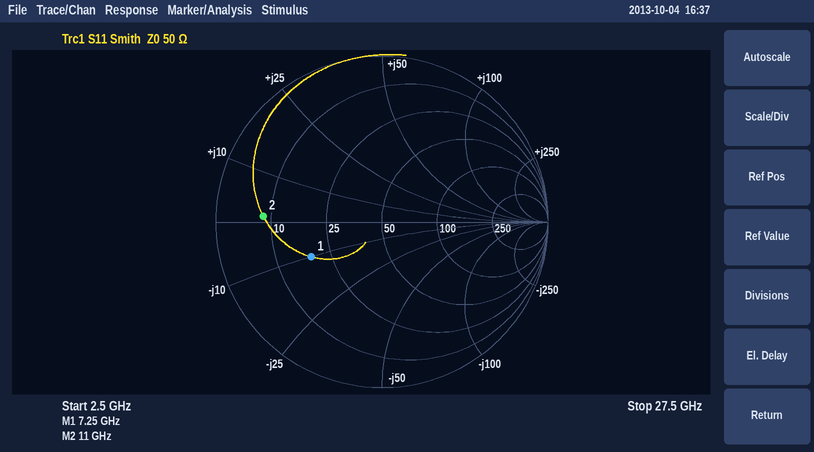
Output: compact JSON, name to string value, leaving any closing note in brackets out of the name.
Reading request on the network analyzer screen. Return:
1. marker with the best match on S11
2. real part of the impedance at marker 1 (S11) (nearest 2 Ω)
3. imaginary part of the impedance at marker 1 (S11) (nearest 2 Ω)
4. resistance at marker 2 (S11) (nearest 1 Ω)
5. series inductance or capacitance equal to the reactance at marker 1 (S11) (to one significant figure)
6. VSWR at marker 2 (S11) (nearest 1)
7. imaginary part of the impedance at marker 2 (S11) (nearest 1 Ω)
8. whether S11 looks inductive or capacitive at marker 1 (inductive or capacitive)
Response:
{"marker with the best match on S11": "marker 1", "real part of the impedance at marker 1 (S11)": "18 Ω", "imaginary part of the impedance at marker 1 (S11)": "-10 Ω", "resistance at marker 2 (S11)": "8 Ω", "series inductance or capacitance equal to the reactance at marker 1 (S11)": "2 pF", "VSWR at marker 2 (S11)": "6", "imaginary part of the impedance at marker 2 (S11)": "+1 Ω", "whether S11 looks inductive or capacitive at marker 1": "capacitive"}
